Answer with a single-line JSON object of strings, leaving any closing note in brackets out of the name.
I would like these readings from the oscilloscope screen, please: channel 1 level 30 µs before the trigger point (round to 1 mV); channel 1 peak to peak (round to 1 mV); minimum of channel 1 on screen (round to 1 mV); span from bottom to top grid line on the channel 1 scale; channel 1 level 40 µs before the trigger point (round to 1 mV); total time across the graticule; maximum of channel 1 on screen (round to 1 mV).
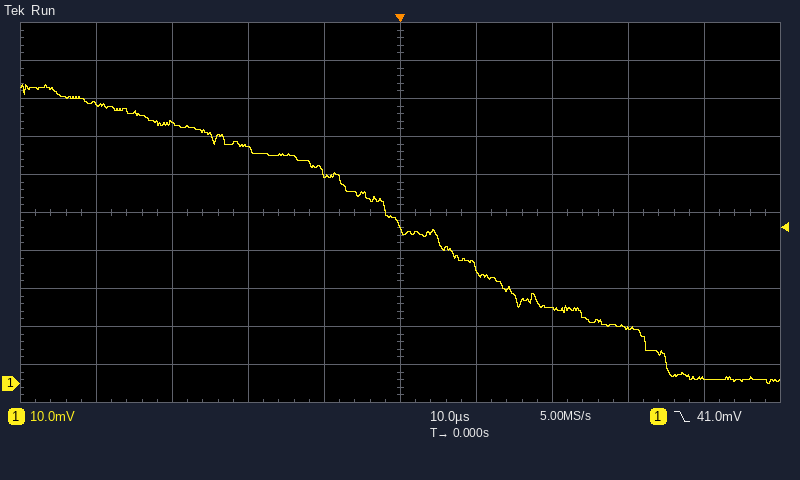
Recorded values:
{"channel 1 level 30 µs before the trigger point": "69 mV", "channel 1 peak to peak": "79 mV", "minimum of channel 1 on screen": "0 mV", "span from bottom to top grid line on the channel 1 scale": "100 mV", "channel 1 level 40 µs before the trigger point": "74 mV", "total time across the graticule": "100 µs", "maximum of channel 1 on screen": "79 mV"}
